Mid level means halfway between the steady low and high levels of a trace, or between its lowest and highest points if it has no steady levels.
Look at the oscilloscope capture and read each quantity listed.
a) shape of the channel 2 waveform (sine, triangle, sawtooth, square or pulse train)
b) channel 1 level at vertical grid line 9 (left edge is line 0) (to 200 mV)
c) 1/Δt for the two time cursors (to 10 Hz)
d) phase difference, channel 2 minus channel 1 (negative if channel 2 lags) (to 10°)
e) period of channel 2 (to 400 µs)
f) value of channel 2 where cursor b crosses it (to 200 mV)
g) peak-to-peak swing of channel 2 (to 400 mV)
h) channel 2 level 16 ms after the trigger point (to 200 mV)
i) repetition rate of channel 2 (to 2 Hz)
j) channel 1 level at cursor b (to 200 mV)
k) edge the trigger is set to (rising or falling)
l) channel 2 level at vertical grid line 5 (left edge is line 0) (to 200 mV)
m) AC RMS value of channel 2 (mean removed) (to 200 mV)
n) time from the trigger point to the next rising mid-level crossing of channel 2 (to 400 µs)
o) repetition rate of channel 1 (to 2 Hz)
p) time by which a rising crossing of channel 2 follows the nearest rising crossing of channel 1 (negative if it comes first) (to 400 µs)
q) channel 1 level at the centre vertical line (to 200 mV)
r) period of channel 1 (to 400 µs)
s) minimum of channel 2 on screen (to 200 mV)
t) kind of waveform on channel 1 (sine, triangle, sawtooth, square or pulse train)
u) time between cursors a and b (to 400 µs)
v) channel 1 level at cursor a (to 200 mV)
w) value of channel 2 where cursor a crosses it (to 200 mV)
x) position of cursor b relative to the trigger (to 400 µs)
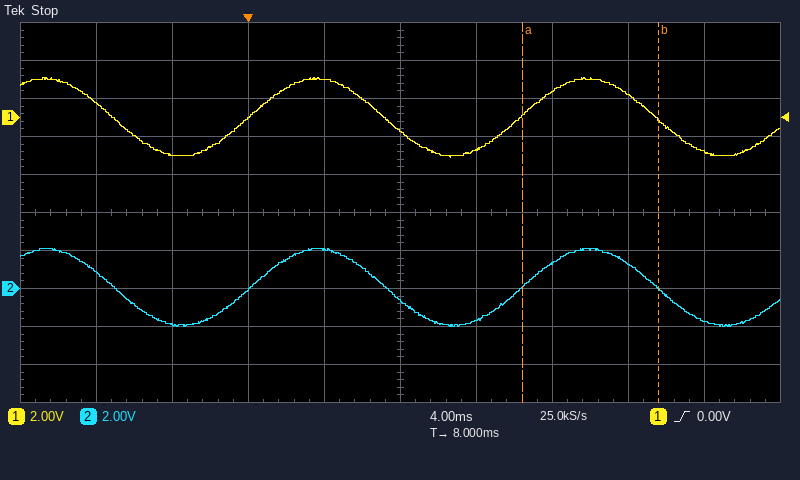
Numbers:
sine
-1.8 V
140 Hz
0°
14.4 ms
0.0 V
4.0 V
1.4 V
70 Hz
-200 mV
rising
-600 mV
1.4 V
14.4 ms
70 Hz
0.0 ms
-800 mV
14.4 ms
-2.0 V
sine
7.2 ms
200 mV
0.0 V
+21.6 ms
